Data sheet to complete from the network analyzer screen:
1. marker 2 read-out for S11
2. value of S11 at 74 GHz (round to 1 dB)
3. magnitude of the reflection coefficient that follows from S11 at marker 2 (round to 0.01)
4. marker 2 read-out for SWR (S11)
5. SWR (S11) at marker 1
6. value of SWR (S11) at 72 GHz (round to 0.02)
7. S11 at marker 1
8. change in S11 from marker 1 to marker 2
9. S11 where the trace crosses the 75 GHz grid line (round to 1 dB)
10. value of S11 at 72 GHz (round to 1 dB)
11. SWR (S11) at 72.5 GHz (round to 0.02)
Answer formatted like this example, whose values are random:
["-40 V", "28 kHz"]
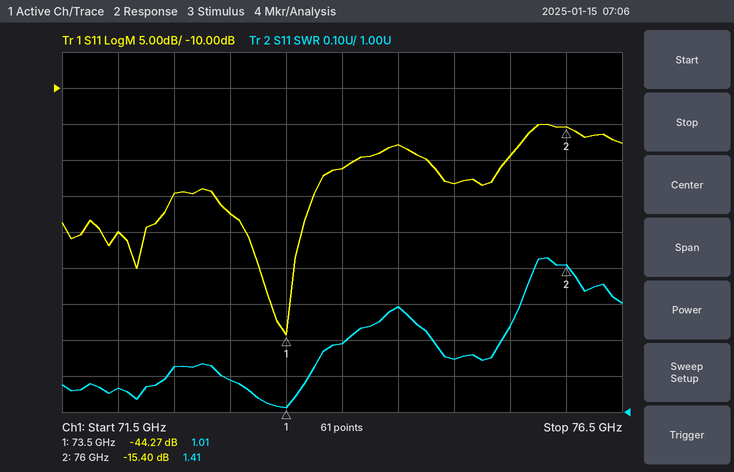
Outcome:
["-15.40 dB", "-21 dB", "0.17", "1.41", "1.01", "1.06", "-44.27 dB", "28.87 dB", "-23 dB", "-30 dB", "1.12"]
